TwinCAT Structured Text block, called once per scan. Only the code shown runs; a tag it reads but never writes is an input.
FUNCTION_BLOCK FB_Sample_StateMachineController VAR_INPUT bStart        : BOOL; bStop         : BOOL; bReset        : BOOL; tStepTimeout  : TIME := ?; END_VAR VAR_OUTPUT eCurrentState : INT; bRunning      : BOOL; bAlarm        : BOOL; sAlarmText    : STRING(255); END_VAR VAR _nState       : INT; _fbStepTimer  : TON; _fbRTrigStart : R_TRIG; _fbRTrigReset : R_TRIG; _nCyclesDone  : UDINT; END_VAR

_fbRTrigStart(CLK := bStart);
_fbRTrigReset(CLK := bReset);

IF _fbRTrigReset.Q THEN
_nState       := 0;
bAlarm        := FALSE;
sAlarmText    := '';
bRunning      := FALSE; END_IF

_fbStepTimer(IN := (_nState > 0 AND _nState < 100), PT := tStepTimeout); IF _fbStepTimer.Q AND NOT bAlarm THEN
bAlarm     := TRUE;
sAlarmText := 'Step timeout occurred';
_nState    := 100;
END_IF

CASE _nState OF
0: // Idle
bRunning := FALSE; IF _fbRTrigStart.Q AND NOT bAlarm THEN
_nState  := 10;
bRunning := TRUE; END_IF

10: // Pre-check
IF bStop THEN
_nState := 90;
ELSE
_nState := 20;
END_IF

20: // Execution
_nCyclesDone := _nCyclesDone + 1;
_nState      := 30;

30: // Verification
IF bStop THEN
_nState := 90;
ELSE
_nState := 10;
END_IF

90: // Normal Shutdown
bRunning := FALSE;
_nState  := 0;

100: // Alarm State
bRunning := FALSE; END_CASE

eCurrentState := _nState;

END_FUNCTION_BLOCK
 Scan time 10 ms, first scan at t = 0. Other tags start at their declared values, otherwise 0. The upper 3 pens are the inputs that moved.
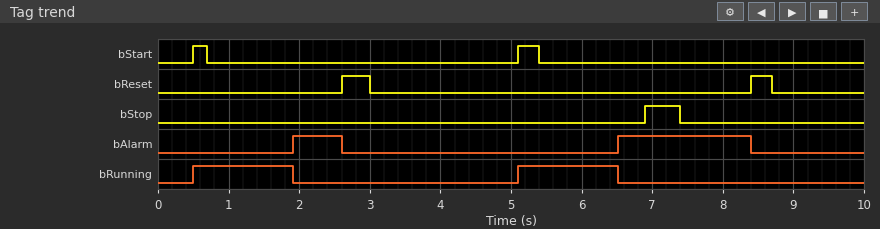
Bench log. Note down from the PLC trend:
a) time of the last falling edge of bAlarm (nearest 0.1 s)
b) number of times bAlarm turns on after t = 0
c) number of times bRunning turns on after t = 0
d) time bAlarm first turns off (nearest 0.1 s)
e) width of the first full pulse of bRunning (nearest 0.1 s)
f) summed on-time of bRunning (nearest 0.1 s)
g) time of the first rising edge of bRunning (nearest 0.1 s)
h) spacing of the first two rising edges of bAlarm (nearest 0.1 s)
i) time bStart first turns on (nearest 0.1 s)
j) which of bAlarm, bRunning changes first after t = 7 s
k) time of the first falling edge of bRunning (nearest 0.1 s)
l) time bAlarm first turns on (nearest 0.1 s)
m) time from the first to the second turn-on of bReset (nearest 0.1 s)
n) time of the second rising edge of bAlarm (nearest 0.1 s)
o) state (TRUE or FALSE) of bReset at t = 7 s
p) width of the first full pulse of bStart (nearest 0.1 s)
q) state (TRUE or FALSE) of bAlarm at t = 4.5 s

8.4 s
2
2
2.6 s
1.4 s
2.8 s
0.5 s
4.6 s
0.5 s
bAlarm
1.9 s
1.9 s
5.8 s
6.5 s
FALSE
0.2 s
FALSE
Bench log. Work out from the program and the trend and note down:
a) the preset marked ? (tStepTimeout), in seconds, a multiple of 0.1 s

1.4 s
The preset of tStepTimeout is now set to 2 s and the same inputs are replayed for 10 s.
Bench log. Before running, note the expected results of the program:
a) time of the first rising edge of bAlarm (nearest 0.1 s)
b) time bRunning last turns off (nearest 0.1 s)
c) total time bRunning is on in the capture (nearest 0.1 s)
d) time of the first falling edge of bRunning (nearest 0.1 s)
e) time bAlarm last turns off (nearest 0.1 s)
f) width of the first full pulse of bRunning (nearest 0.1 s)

2.5 s
6.9 s
3.8 s
2.5 s
2.6 s
2.0 s
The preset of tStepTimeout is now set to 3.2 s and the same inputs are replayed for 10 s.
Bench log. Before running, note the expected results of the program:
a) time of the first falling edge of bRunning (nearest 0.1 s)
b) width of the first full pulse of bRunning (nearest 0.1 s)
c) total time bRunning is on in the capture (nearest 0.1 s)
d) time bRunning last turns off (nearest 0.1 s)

2.6 s
2.1 s
3.9 s
6.9 s
